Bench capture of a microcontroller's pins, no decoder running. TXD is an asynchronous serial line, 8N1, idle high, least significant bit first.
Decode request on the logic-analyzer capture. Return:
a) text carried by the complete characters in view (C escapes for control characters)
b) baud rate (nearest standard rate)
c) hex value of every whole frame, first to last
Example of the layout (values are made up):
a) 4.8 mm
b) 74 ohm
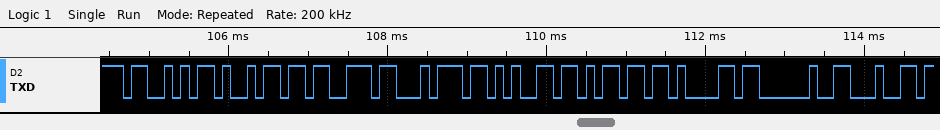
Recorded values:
a) "Sistema d"
b) 9600 baud
c) 0x53 0x69 0x73 0x74 0x65 0x6D 0x61 0x20 0x64
